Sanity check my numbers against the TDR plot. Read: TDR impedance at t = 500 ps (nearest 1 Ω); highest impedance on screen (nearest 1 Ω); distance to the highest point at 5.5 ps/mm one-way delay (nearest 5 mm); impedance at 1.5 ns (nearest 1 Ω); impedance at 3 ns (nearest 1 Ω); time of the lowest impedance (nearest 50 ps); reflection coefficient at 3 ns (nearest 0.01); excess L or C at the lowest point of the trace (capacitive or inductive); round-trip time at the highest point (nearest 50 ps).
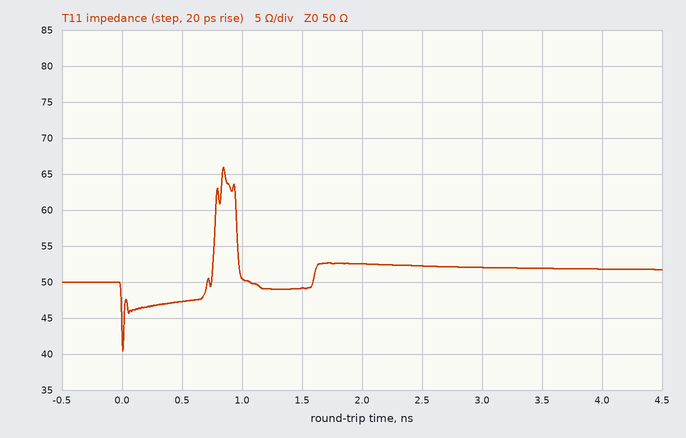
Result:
47 Ω
66 Ω
75 mm
49 Ω
52 Ω
0 ps
+0.02
capacitive
850 ps
